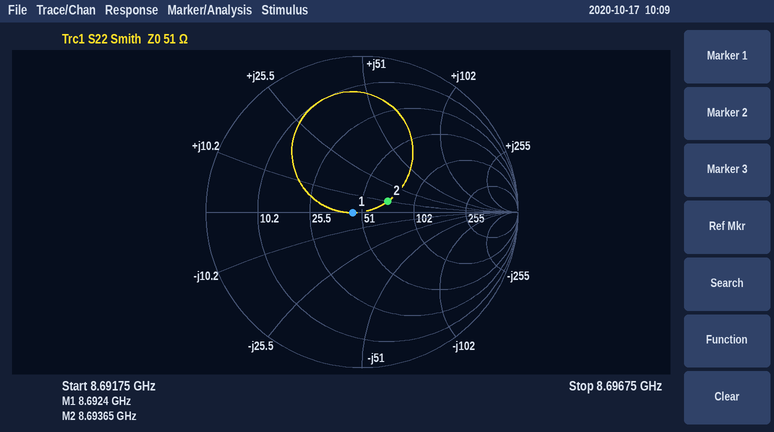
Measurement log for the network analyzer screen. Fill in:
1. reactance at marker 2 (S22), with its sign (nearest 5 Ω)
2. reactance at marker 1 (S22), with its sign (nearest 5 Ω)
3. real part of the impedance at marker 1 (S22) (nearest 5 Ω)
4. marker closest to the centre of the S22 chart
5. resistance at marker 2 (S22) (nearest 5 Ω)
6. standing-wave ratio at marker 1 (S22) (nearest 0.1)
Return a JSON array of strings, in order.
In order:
["+10 Ω", "0 Ω", "45 Ω", "marker 1", "70 Ω", "1.1"]
